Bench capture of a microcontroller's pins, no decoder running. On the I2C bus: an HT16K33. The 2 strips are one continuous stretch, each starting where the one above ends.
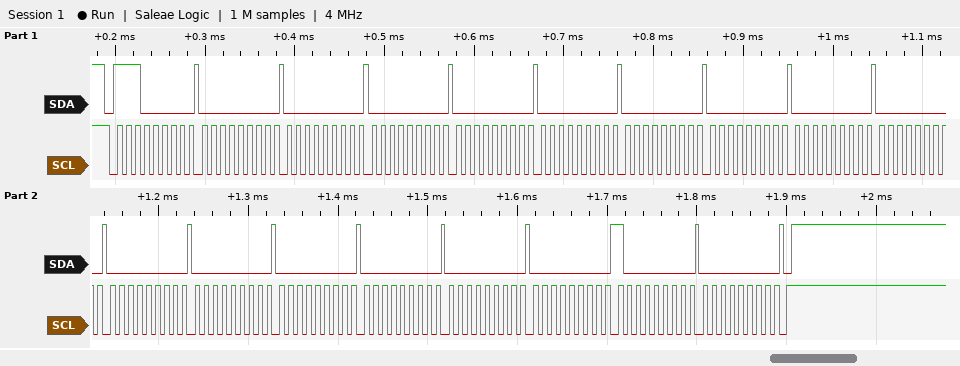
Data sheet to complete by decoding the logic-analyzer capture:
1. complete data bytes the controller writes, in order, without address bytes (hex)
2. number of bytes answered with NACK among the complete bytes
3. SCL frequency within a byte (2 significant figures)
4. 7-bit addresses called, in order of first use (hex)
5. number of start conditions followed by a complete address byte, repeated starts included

00 00 00 00 00 00 00 00 00 00 00 00 00 00 00 80 00
0
100 kHz
0x70
1
